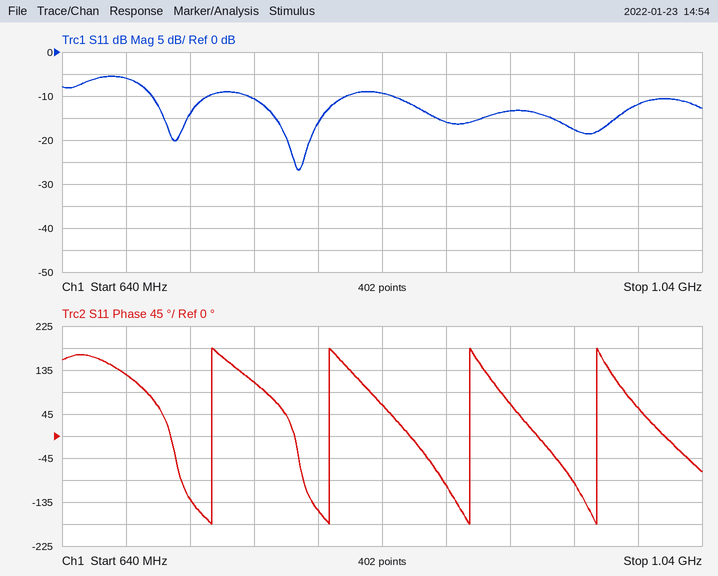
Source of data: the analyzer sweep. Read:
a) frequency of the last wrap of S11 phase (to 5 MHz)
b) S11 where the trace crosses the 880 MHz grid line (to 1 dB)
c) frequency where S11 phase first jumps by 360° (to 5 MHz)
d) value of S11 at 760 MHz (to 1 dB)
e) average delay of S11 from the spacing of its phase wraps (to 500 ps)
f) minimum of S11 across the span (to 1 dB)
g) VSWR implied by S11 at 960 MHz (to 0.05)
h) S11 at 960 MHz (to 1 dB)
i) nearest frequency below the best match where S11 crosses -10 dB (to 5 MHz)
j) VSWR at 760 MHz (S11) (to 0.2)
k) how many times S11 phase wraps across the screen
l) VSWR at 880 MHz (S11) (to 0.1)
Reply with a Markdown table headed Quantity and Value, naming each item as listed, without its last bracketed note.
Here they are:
| Quantity | Value |
|---|---|
| frequency of the last wrap of S11 phase | 975 MHz |
| S11 where the trace crosses the 880 MHz grid line | -16 dB |
| frequency where S11 phase first jumps by 360° | 735 MHz |
| value of S11 at 760 MHz | -11 dB |
| average delay of S11 from the spacing of its phase wraps | 12.5 ns |
| minimum of S11 across the span | -27 dB |
| VSWR implied by S11 at 960 MHz | 1.30 |
| S11 at 960 MHz | -18 dB |
| nearest frequency below the best match where S11 crosses -10 dB | 755 MHz |
| VSWR at 760 MHz (S11) | 1.8 |
| how many times S11 phase wraps across the screen | 4 |
| VSWR at 880 MHz (S11) | 1.4 |
